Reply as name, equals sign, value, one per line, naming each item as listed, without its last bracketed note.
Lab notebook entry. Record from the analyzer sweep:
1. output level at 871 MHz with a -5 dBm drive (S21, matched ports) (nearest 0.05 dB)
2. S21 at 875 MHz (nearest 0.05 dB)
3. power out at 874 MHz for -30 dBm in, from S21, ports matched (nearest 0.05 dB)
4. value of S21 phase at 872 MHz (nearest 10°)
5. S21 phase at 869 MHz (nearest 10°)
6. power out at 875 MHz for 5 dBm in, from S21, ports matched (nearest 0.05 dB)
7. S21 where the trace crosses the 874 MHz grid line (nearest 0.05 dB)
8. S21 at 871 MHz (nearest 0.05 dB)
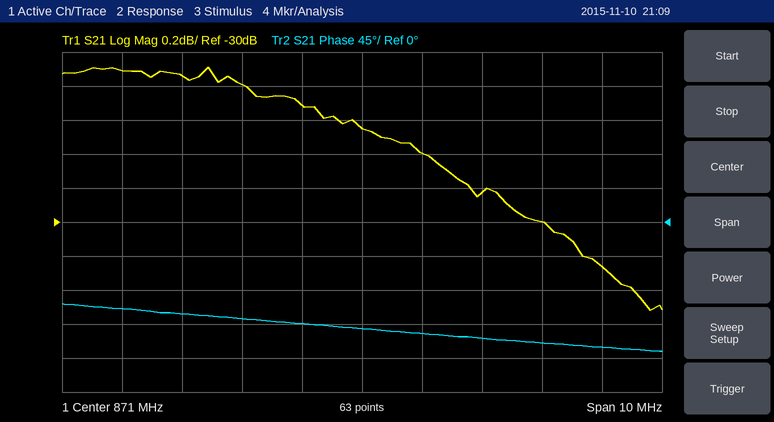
output level at 871 MHz with a -5 dBm drive (S21, matched ports) = -34.45 dBm
S21 at 875 MHz = -30.25 dB
power out at 874 MHz for -30 dBm in, from S21, ports matched = -60.00 dBm
value of S21 phase at 872 MHz = -150°
S21 phase at 869 MHz = -130°
power out at 875 MHz for 5 dBm in, from S21, ports matched = -25.25 dBm
S21 where the trace crosses the 874 MHz grid line = -30.00 dB
S21 at 871 MHz = -29.45 dB
